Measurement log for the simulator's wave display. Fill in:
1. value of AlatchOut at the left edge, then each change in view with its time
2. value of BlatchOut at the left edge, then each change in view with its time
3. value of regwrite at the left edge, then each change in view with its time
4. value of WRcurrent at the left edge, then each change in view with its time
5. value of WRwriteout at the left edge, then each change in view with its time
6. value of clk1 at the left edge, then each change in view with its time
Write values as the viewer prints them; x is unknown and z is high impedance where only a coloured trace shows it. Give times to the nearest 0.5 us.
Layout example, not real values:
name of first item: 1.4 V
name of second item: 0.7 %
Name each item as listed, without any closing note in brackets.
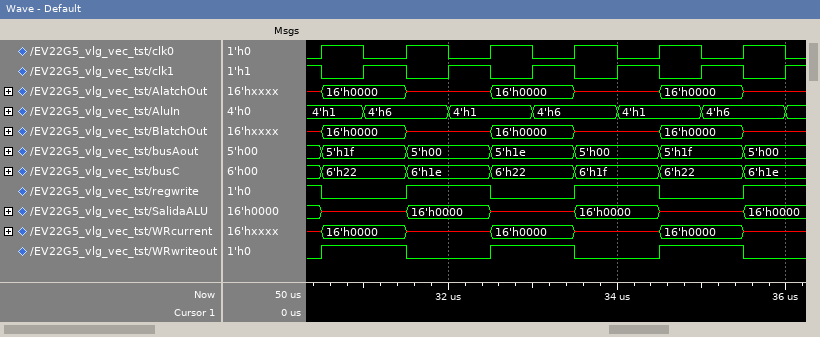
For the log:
value of AlatchOut at the left edge, then each change in view with its time: x, 16'h0000 at 30.5 us, x at 31.5 us, 16'h0000 at 32.5 us, x at 33.5 us, 16'h0000 at 34.5 us, x at 35.5 us
value of BlatchOut at the left edge, then each change in view with its time: x, 16'h0000 at 30.5 us, x at 31.5 us, 16'h0000 at 32.5 us, x at 33.5 us, 16'h0000 at 34.5 us, x at 35.5 us
value of regwrite at the left edge, then each change in view with its time: 1, 0 at 30.5 us, 1 at 31.5 us, 0 at 32.5 us, 1 at 33.5 us, 0 at 34.5 us, 1 at 35.5 us
value of WRcurrent at the left edge, then each change in view with its time: x, 16'h0000 at 30.5 us, x at 31.5 us, 16'h0000 at 32.5 us, x at 33.5 us, 16'h0000 at 34.5 us, x at 35.5 us
value of WRwriteout at the left edge, then each change in view with its time: 0, 1 at 30.5 us, 0 at 31.5 us, 1 at 32.5 us, 0 at 33.5 us, 1 at 34.5 us, 0 at 35.5 us
value of clk1 at the left edge, then each change in view with its time: 1, 0 at 30.5 us, 1 at 31 us, 0 at 31.5 us, 1 at 32 us, 0 at 32.5 us, 1 at 33 us, 0 at 33.5 us, 1 at 34 us, 0 at 34.5 us, 1 at 35 us, 0 at 35.5 us, 1 at 36 us
